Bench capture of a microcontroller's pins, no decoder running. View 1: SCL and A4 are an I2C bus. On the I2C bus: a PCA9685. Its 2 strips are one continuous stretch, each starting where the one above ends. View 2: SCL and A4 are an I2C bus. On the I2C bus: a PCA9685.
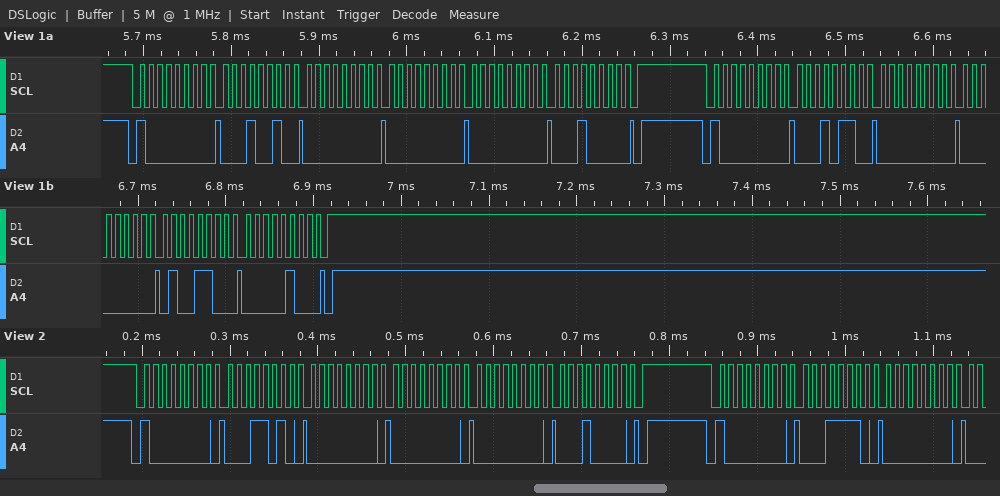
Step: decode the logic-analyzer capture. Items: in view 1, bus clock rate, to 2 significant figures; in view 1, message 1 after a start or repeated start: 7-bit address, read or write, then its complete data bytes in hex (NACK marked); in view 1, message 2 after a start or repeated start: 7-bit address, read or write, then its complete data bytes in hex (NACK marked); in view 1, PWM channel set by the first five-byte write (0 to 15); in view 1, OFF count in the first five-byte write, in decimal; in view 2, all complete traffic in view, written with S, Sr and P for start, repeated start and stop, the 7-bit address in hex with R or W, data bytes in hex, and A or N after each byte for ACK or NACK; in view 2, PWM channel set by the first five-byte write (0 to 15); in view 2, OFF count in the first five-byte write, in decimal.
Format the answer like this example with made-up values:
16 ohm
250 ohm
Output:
100 kHz
0x40 write: 12 00 00 00 10
0x40 write: 16 00 00 4C 04
3
4096
S 40W A 1A A 00 A 00 A 00 A 10 A P S 40W A 1E A 00 A
5
4096
